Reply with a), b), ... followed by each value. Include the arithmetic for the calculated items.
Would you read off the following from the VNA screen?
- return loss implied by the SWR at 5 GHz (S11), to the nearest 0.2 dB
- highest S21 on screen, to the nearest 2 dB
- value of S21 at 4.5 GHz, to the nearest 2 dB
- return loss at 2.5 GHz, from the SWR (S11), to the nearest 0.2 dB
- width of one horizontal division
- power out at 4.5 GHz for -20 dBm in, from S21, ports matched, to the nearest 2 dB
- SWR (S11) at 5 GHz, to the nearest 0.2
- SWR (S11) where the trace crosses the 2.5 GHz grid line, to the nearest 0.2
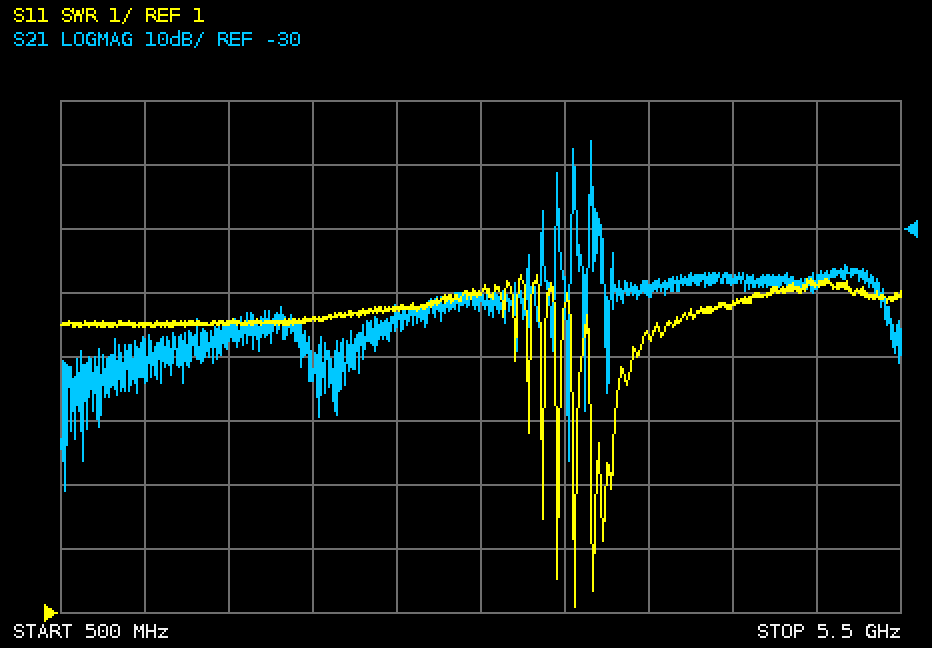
a) −20 log10((6.2 − 1)/(6.2 + 1)) ≈ 2.8 dB
b) -16 dB
c) -38 dB
d) −20 log10((5.8 − 1)/(5.8 + 1)) ≈ 3.0 dB
e) 500 MHz
f) -20 dBm + (-38 dB) = -58 dBm
g) 6.2
h) 5.8
